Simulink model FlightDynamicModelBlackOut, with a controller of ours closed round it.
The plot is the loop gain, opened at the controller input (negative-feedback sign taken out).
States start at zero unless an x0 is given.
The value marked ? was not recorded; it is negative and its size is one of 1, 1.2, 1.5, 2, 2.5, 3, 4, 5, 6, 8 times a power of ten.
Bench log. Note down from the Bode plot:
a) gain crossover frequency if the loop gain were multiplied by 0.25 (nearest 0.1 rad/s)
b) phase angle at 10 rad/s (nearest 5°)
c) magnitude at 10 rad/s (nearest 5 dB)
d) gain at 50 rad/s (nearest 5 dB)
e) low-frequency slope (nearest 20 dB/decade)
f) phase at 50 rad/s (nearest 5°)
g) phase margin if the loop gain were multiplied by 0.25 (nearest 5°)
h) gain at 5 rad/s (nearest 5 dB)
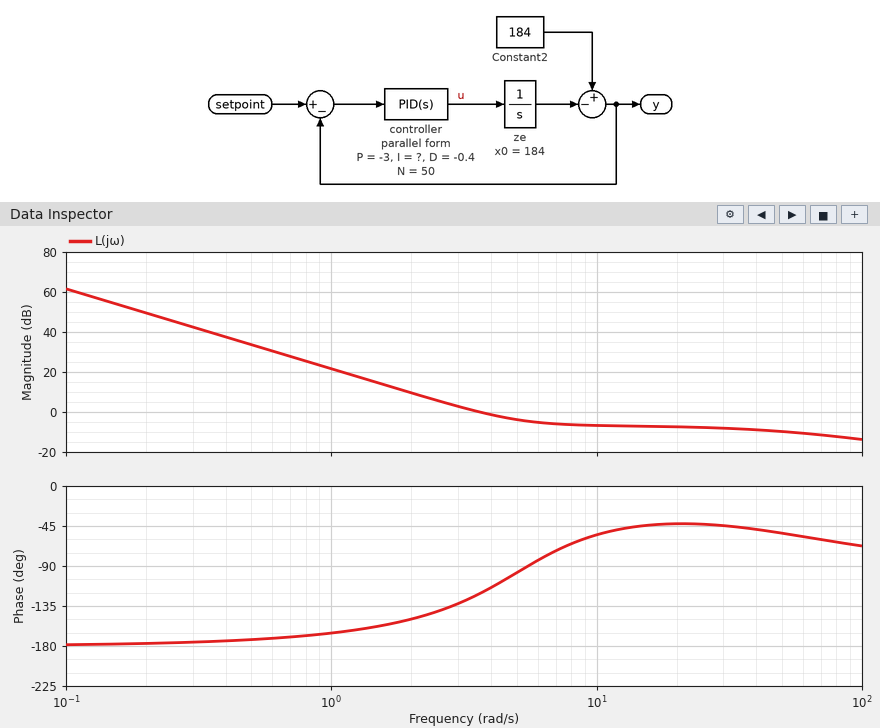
1.7 rad/s
-55°
-5 dB
-10 dB
-40 dB/decade
-55°
25°
-5 dB
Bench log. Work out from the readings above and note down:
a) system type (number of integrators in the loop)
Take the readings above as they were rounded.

2
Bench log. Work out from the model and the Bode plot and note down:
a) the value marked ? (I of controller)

-12
